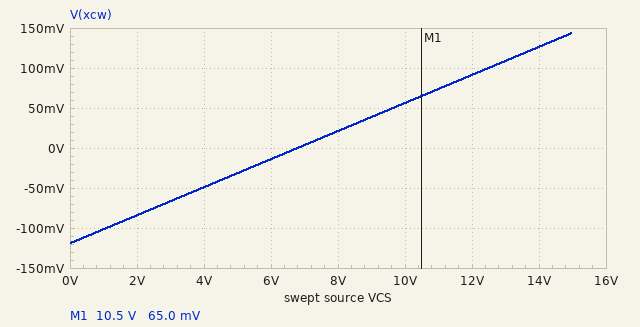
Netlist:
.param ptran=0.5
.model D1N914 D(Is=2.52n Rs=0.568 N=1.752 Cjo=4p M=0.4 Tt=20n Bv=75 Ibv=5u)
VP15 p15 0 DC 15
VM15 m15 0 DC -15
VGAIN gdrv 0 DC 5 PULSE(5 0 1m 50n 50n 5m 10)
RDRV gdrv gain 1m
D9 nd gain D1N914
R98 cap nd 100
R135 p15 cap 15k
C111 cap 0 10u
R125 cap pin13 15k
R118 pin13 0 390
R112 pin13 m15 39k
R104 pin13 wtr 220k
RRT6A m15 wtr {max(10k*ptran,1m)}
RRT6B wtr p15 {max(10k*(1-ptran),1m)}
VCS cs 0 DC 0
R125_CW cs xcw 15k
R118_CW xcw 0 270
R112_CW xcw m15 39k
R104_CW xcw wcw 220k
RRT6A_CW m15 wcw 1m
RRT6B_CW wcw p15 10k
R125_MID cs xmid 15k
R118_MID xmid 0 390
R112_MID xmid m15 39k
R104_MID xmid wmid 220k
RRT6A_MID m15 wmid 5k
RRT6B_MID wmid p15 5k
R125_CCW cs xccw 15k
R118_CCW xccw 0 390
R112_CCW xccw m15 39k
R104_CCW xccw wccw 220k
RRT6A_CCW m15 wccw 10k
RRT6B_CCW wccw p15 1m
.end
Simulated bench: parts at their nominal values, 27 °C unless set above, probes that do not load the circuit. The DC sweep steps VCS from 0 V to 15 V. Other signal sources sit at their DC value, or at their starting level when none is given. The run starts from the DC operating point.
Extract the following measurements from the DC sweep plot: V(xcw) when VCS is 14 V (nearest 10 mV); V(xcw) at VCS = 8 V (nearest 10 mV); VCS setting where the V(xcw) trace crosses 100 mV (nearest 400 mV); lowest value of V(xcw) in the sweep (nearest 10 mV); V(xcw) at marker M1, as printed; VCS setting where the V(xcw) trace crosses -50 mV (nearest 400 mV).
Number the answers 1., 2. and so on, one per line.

1. 130 mV
2. 20 mV
3. 12.4 V
4. -120 mV
5. 65.0 mV
6. 4.0 V
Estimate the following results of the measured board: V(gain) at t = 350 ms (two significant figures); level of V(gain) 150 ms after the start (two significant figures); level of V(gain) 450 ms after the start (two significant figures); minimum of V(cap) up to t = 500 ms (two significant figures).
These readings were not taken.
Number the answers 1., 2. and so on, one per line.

1. 5.0 V
2. 5.0 V
3. 5.0 V
4. 740 mV
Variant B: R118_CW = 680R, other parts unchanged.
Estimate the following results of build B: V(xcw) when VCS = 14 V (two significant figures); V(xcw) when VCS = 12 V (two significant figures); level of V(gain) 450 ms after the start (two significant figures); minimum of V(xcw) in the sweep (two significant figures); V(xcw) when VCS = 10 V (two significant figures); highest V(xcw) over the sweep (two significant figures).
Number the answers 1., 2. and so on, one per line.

1. 310 mV
2. 220 mV
3. 5.0 V
4. -290 mV
5. 140 mV
6. 350 mV
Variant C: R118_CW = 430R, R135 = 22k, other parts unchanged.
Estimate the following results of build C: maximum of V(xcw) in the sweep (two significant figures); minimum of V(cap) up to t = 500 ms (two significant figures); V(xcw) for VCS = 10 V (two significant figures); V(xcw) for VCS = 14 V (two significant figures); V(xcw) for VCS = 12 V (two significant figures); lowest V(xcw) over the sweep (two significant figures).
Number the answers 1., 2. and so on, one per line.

1. 230 mV
2. 700 mV
3. 88 mV
4. 200 mV
5. 140 mV
6. -190 mV
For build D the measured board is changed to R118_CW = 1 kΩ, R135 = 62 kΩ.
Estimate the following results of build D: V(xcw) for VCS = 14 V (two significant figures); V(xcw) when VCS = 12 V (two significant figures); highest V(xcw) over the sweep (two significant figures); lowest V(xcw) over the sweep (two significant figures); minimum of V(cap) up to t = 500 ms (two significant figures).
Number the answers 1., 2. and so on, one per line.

1. 440 mV
2. 320 mV
3. 500 mV
4. -410 mV
5. 610 mV
